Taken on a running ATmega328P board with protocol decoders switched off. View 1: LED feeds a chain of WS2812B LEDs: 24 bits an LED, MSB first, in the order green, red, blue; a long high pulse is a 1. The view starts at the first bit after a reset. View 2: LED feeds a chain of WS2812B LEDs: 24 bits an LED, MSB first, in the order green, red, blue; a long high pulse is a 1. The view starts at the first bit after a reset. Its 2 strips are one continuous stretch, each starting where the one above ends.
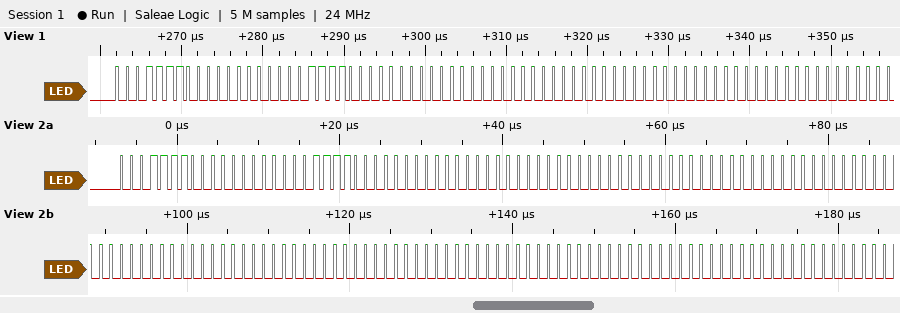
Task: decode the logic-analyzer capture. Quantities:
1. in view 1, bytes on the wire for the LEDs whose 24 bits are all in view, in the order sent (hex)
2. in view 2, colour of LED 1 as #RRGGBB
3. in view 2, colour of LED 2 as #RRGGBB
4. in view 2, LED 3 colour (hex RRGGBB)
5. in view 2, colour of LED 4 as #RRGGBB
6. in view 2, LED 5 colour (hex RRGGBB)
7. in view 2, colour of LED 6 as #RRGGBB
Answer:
1E 00 1E 00 00 00 00 00 00
#001E1E
#000000
#000000
#000000
#000000
#000000
